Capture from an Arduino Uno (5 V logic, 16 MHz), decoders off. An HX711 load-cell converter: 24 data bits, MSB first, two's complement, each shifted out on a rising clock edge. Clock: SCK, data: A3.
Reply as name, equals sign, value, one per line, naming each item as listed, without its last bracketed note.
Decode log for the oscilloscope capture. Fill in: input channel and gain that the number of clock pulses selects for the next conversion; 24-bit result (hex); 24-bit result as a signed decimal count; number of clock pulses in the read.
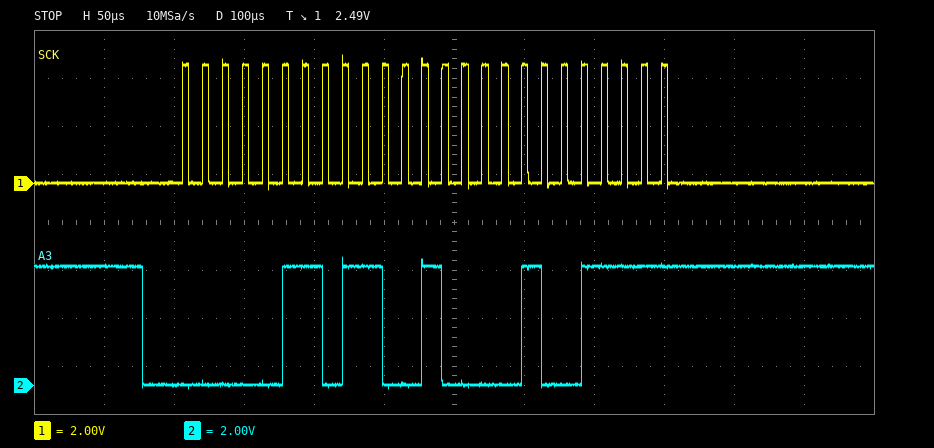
input channel and gain that the number of clock pulses selects for the next conversion = channel A, gain 128
24-bit result = 0x06C84F
24-bit result as a signed decimal count = 444495
number of clock pulses in the read = 25
